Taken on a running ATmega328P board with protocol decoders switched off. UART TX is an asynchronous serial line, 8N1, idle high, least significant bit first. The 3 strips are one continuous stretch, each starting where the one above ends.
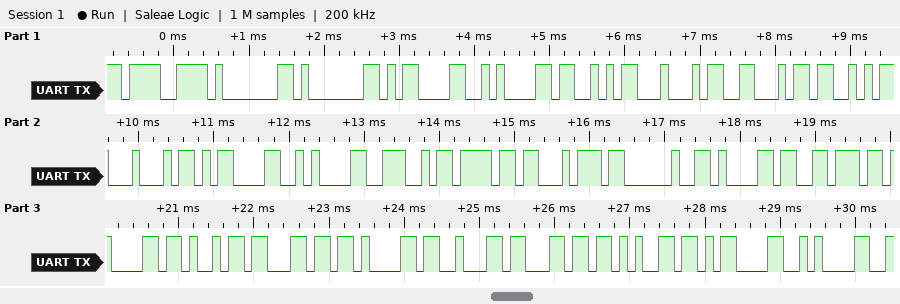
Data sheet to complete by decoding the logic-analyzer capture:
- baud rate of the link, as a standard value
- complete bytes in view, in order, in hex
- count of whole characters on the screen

9600 baud
CF 01 01 0D 0A 53 44 46 53 44 0D 0A 4E 6F 74 20 61 76 61 69 6C 61 62 6C 65 0D 0A
27
